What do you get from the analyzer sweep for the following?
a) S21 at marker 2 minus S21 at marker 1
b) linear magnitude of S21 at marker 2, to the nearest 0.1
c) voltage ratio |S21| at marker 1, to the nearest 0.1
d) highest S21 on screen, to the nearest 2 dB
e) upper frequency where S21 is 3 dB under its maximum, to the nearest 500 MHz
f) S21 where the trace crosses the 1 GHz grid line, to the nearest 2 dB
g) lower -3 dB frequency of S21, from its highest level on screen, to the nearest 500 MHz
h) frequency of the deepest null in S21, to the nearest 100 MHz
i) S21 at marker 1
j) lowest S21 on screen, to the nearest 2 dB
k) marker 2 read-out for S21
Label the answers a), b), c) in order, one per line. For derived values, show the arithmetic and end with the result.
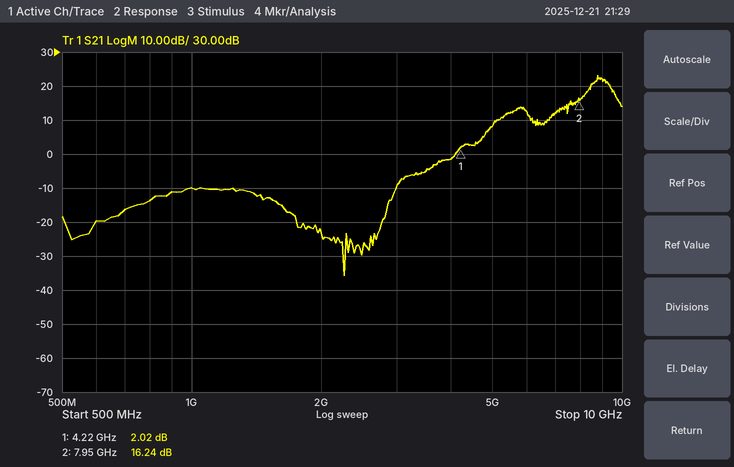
a) 16.24 − (2.02) = 14.22 dB
b) 10^(16.24/20) ≈ 6.5
c) 10^(2.02/20) ≈ 1.3
d) 24 dB
e) 9.5 GHz
f) -10 dB
g) 8.5 GHz
h) 2.3 GHz
i) 2.02 dB
j) -36 dB
k) 16.24 dB
